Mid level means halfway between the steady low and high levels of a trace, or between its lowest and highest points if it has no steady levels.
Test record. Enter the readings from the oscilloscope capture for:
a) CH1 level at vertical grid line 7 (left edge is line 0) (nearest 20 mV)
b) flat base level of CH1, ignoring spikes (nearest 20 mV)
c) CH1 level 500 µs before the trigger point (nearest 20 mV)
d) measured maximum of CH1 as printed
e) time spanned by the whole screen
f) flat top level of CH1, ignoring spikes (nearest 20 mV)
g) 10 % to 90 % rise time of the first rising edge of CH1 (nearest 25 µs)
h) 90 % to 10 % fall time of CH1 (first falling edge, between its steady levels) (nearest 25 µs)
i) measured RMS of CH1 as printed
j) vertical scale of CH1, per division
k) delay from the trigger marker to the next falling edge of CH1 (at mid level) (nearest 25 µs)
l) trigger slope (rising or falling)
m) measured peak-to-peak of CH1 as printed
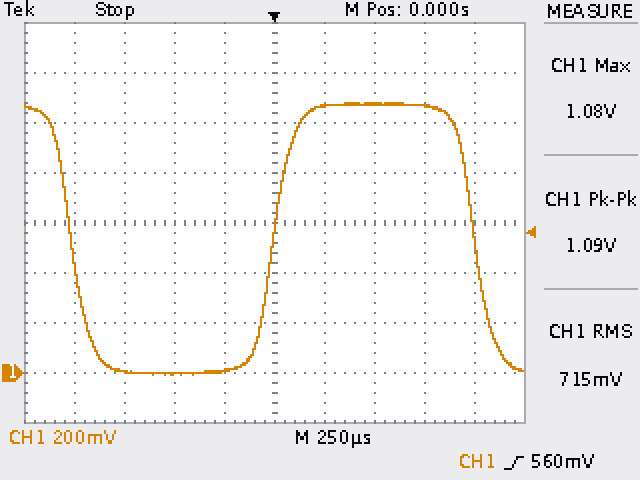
1.08 V
0 mV
0 mV
1.08 V
2.5 ms
1.08 V
200 µs
200 µs
715 mV
200 mV
1.000 ms
rising
1.09 V
